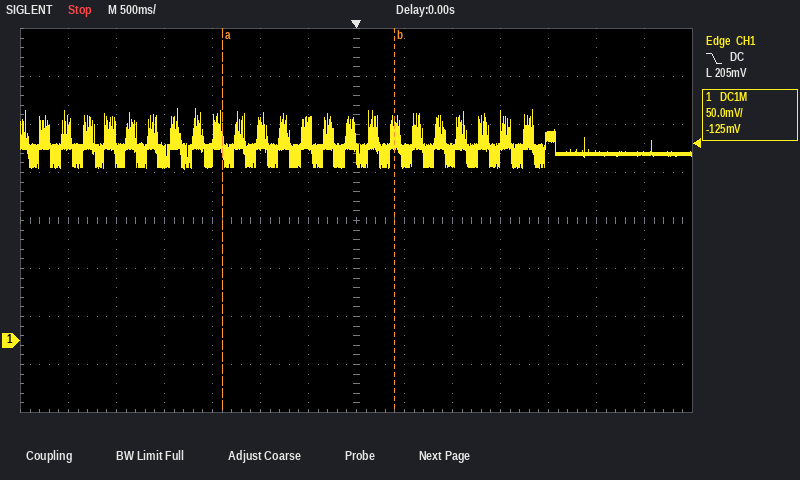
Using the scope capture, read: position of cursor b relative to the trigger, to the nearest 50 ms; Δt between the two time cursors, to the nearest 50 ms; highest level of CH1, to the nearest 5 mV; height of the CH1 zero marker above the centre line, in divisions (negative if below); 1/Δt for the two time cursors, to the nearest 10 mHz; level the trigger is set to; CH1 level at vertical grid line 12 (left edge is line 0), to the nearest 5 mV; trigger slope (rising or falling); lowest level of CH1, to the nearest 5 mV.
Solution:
+400 ms
1.80 s
240 mV
-2.5 div
560 mHz
205 mV
195 mV
falling
180 mV
